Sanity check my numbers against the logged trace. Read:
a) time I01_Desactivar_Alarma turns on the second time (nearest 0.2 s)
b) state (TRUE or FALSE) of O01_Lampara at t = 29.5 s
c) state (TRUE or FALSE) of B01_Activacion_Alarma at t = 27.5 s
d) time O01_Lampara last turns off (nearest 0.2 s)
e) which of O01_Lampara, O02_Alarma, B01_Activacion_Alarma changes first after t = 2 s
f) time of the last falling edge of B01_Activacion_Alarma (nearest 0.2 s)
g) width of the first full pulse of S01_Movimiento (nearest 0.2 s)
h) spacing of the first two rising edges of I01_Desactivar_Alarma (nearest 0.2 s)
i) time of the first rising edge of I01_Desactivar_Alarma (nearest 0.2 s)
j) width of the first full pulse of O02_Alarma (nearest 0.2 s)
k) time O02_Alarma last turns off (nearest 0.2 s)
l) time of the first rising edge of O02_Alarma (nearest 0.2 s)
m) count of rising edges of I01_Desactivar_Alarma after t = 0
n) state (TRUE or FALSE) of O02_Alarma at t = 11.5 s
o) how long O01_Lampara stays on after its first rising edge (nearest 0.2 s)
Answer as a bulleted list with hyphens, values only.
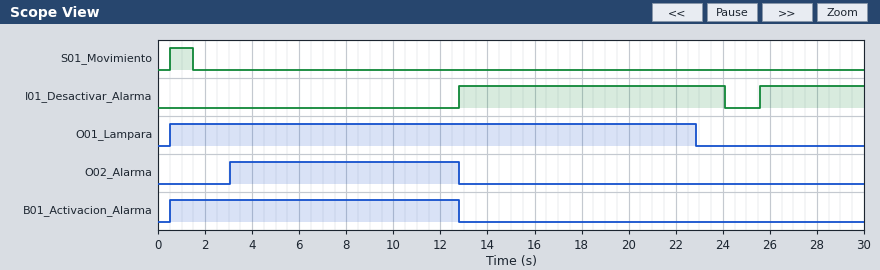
- 25.6 s
- FALSE
- FALSE
- 22.8 s
- O02_Alarma
- 12.8 s
- 1.0 s
- 12.8 s
- 12.8 s
- 9.8 s
- 12.8 s
- 3.0 s
- 2
- TRUE
- 22.4 s
